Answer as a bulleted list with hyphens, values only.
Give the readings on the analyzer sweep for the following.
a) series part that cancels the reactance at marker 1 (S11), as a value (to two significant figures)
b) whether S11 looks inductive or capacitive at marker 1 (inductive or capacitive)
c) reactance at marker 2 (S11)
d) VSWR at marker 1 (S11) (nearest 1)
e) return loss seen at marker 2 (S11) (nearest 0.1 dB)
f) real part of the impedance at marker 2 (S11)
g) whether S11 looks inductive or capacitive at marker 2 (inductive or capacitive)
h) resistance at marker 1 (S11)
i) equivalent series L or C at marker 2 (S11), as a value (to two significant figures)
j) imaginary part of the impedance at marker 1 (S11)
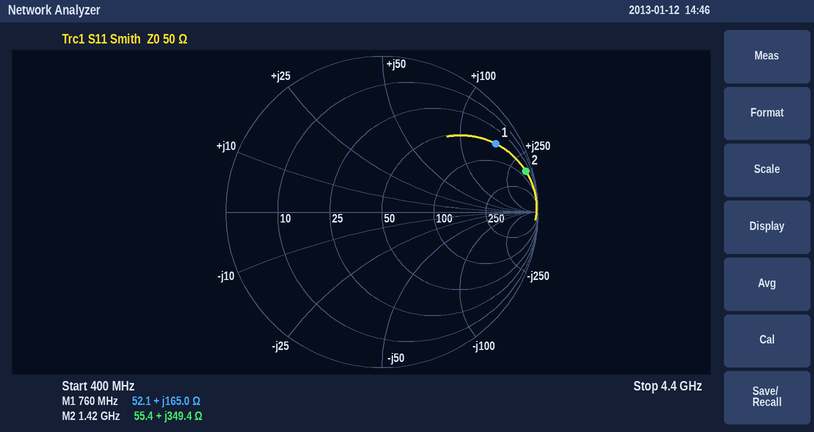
- 1.3 pF
- inductive
- +349.4 Ω
- 12
- 0.4 dB
- 55.4 Ω
- inductive
- 52.1 Ω
- 39 nH
- +165.0 Ω
